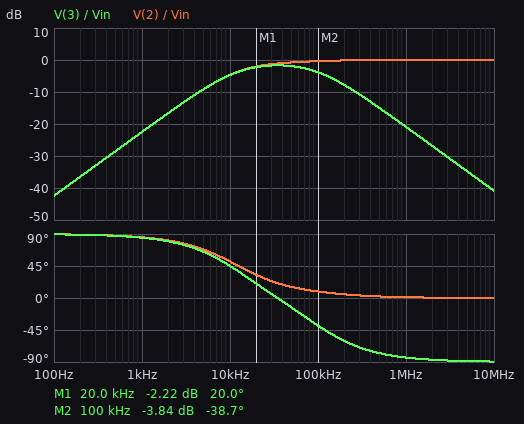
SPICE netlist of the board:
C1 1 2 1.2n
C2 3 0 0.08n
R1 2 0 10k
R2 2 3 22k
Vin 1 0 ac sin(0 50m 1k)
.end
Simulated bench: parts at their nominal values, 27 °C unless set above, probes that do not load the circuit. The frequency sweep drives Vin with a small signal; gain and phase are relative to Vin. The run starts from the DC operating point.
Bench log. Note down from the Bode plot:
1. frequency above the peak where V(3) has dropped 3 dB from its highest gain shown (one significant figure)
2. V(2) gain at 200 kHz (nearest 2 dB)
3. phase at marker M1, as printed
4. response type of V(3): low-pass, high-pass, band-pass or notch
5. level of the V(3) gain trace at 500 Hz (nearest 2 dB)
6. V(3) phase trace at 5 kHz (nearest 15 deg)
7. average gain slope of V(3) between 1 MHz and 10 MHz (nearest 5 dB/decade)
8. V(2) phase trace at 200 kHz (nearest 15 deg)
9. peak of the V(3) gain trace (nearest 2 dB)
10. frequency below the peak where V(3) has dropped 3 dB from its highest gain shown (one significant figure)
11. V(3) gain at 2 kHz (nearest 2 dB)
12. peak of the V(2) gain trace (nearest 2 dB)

100 kHz
0 dB
20.0 deg
band-pass
-28 dB
60 deg
-20 dB/decade
0 deg
-2 dB
10 kHz
-16 dB
0 dB
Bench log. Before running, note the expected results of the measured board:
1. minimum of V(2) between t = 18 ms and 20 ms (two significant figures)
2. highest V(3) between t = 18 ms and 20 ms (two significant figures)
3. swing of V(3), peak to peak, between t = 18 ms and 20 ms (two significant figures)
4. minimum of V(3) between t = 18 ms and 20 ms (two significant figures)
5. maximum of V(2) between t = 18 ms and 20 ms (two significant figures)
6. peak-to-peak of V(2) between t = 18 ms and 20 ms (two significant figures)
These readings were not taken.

-3.8 mV
3.8 mV
7.5 mV
-3.8 mV
3.8 mV
7.5 mV
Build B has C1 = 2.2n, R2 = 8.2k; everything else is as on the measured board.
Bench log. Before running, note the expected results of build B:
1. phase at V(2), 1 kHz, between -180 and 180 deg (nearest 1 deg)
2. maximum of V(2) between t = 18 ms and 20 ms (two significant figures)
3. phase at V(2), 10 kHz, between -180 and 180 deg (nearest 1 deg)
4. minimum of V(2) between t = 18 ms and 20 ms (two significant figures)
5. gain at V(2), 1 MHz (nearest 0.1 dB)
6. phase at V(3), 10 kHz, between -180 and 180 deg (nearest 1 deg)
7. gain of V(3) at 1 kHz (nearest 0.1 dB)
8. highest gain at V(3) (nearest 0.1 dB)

82 deg
6.8 mV
35 deg
-6.8 mV
0 dB
33 deg
-17.3 dB
-0.6 dB
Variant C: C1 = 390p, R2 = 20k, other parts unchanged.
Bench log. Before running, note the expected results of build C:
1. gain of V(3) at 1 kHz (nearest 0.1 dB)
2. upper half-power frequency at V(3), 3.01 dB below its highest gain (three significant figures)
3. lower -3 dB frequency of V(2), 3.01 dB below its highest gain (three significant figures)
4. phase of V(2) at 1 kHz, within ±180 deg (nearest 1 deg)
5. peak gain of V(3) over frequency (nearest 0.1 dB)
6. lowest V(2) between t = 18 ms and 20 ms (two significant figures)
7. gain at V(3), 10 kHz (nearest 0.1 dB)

-32.2 dB
183 kHz
56.1 kHz
88 deg
-4.2 dB
-1.2 mV
-12.7 dB
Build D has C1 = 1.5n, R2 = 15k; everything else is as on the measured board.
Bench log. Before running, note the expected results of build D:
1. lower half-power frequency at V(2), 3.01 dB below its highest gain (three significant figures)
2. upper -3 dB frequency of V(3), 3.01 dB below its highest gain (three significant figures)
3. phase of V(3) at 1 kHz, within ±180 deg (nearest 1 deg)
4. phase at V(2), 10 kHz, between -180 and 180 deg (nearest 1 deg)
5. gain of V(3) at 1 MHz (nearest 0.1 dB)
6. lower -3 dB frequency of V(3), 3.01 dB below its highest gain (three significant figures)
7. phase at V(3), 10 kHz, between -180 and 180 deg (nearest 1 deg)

11.3 kHz
159 kHz
84 deg
45 deg
-17.6 dB
8.84 kHz
41 deg
